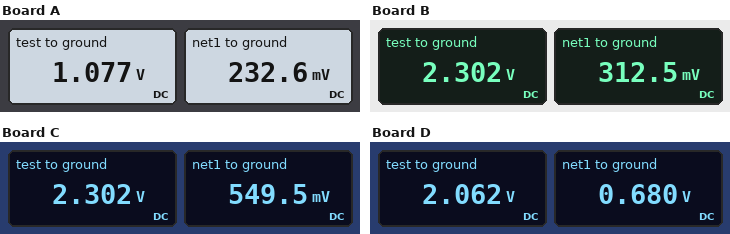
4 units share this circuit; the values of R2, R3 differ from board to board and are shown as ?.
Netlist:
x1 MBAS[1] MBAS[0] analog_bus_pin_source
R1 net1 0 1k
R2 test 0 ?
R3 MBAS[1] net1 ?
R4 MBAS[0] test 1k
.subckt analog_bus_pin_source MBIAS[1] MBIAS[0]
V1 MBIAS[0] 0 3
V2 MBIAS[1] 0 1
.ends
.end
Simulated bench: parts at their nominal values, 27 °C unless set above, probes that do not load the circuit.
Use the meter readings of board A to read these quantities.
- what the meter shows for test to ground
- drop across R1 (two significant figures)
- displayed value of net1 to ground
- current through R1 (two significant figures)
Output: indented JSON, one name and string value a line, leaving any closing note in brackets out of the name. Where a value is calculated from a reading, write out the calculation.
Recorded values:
{
  "what the meter shows for test to ground": "1.077 V",
  "drop across R1": "232.6 mV = 230 mV",
  "displayed value of net1 to ground": "232.6 mV",
  "current through R1": "(232.6 mV) / 1 kΩ = 230 µA"
}
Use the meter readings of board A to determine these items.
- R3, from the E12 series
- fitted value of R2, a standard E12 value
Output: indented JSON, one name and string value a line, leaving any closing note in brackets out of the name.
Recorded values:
{
  "R3, from the E12 series": "3.3 kΩ",
  "fitted value of R2, a standard E12 value": "560 Ω"
}
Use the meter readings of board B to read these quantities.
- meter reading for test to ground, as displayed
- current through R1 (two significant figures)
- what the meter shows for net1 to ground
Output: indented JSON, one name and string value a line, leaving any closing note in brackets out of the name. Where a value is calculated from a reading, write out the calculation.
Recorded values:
{
  "meter reading for test to ground, as displayed": "2.302 V",
  "current through R1": "(312.5 mV) / 1 kΩ = 310 µA",
  "what the meter shows for net1 to ground": "312.5 mV"
}
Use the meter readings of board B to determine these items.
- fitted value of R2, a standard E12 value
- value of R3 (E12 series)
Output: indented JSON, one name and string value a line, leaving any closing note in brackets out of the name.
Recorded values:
{
  "fitted value of R2, a standard E12 value": "3.3 kΩ",
  "value of R3": "2.2 kΩ"
}
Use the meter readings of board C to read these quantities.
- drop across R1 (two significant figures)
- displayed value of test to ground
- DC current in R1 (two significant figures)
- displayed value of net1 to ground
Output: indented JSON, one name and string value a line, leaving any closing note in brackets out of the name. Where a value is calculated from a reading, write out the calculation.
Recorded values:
{
  "drop across R1": "549.5 mV = 550 mV",
  "displayed value of test to ground": "2.302 V",
  "DC current in R1": "(549.5 mV) / 1 kΩ = 550 µA",
  "displayed value of net1 to ground": "549.5 mV"
}
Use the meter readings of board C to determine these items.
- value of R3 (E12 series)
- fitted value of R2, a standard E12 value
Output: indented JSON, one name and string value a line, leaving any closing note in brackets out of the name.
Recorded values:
{
  "value of R3": "820 Ω",
  "fitted value of R2, a standard E12 value": "3.3 kΩ"
}
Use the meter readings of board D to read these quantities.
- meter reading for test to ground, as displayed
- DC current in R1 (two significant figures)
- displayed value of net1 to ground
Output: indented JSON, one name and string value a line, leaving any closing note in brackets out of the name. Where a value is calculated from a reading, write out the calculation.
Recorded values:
{
  "meter reading for test to ground, as displayed": "2.062 V",
  "DC current in R1": "(680 mV) / 1 kΩ = 680 µA",
  "displayed value of net1 to ground": "0.680 V"
}
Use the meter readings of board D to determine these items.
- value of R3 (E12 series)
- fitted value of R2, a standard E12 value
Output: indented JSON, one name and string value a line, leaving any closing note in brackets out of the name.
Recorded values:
{
  "value of R3": "470 Ω",
  "fitted value of R2, a standard E12 value": "2.2 kΩ"
}
